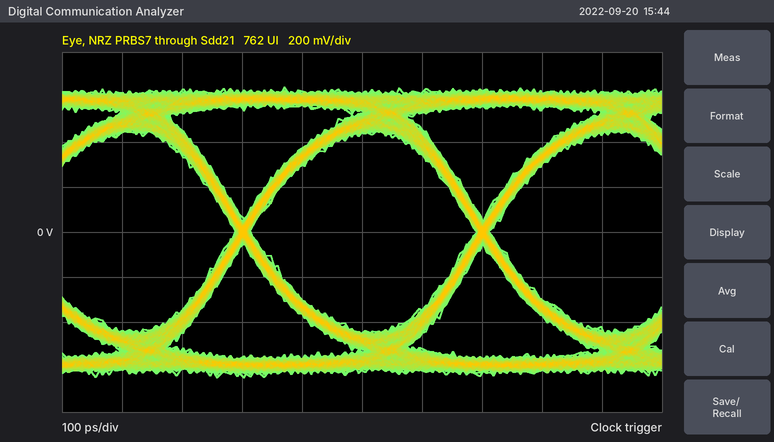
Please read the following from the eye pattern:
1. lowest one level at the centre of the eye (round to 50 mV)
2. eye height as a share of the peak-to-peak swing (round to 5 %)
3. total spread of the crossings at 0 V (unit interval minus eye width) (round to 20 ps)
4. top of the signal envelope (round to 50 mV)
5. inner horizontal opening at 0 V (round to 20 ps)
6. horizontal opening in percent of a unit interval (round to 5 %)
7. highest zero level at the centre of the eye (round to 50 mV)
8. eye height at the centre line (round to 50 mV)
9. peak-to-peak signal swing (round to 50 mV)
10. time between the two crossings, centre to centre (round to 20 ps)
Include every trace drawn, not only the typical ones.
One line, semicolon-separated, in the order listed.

450 mV; 70 %; 20 ps; 650 mV; 380 ps; 95 %; -450 mV; 900 mV; 1.30 V; 400 ps
